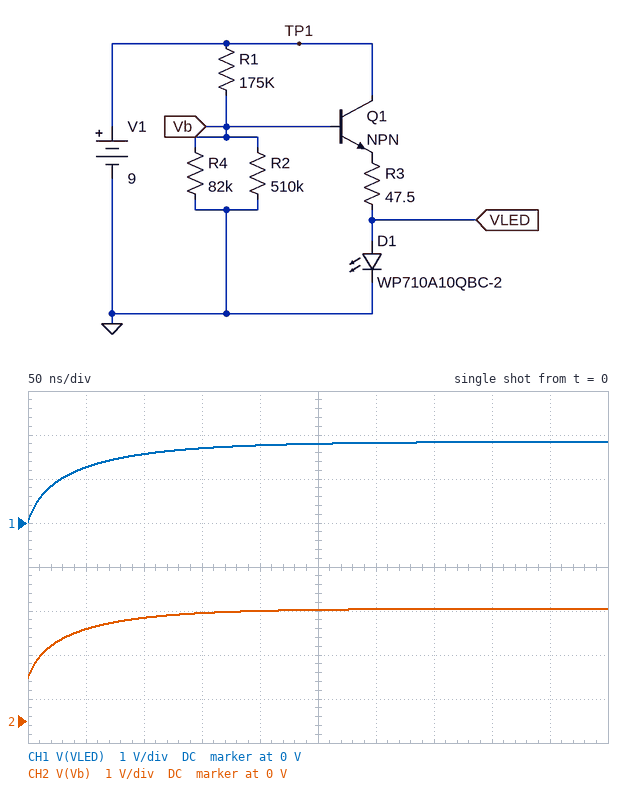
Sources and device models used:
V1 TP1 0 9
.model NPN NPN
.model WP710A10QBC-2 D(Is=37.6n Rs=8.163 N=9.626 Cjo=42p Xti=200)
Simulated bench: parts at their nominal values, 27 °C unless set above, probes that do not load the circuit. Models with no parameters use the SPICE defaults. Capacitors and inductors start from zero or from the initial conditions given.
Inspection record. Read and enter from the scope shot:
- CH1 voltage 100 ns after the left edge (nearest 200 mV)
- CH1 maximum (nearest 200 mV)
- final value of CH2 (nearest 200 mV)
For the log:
1.6 V
1.8 V
2.6 V
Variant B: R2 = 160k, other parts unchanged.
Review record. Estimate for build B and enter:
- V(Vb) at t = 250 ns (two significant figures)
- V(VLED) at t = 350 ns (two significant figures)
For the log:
2.1 V
1.4 V
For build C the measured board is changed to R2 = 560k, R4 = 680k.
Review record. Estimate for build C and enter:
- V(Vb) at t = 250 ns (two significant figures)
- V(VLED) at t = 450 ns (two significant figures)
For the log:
3.6 V
2.7 V
